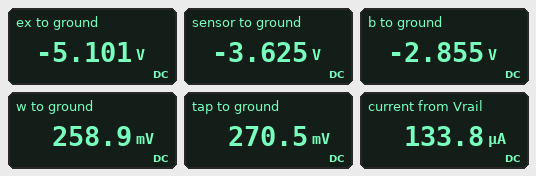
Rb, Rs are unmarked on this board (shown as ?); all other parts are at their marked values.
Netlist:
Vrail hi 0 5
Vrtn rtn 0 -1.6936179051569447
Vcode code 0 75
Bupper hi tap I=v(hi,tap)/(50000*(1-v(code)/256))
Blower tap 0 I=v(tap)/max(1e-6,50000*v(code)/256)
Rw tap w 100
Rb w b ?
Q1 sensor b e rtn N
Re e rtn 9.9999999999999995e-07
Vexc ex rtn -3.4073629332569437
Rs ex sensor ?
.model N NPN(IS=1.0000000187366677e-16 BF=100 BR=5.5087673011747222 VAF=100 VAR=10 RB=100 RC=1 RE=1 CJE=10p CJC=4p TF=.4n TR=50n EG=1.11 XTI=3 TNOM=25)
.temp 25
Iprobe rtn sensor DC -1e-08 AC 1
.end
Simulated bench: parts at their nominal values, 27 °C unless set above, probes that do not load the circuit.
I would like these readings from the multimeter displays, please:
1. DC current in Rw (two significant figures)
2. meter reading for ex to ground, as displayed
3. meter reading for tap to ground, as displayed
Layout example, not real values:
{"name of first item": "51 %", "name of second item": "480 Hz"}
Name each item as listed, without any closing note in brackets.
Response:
{"DC current in Rw": "120 µA", "meter reading for ex to ground, as displayed": "-5.101 V", "meter reading for tap to ground, as displayed": "270.5 mV"}
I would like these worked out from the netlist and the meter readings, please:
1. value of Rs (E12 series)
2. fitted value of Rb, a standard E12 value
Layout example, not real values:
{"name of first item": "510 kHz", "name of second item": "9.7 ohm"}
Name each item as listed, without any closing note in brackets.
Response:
{"value of Rs": "1.8 kΩ", "fitted value of Rb, a standard E12 value": "27 kΩ"}
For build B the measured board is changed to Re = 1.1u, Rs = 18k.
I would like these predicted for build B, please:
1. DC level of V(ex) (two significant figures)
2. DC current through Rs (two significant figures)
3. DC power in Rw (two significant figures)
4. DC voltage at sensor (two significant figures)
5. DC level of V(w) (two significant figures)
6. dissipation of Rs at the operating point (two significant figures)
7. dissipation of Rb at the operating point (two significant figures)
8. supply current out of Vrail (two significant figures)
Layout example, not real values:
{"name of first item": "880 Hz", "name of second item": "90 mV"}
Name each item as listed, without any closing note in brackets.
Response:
{"DC level of V(ex)": "-5.1 V", "DC current through Rs": "190 µA", "DC power in Rw": "420 nW", "DC voltage at sensor": "-1.7 V", "DC level of V(w)": "790 mV", "dissipation of Rs at the operating point": "640 µW", "dissipation of Rb at the operating point": "110 µW", "supply current out of Vrail": "120 µA"}
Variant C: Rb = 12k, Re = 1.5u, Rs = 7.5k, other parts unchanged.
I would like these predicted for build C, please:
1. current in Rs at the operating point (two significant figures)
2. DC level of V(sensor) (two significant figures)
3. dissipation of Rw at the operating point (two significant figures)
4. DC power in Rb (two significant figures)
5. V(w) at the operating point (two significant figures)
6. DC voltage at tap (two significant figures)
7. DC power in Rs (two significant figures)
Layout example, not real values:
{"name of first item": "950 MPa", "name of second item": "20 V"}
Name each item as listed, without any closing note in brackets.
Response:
{"current in Rs at the operating point": "450 µA", "DC level of V(sensor)": "-1.7 V", "dissipation of Rw at the operating point": "1.2 µW", "DC power in Rb": "140 µW", "V(w) at the operating point": "340 mV", "DC voltage at tap": "350 mV", "DC power in Rs": "1.5 mW"}
